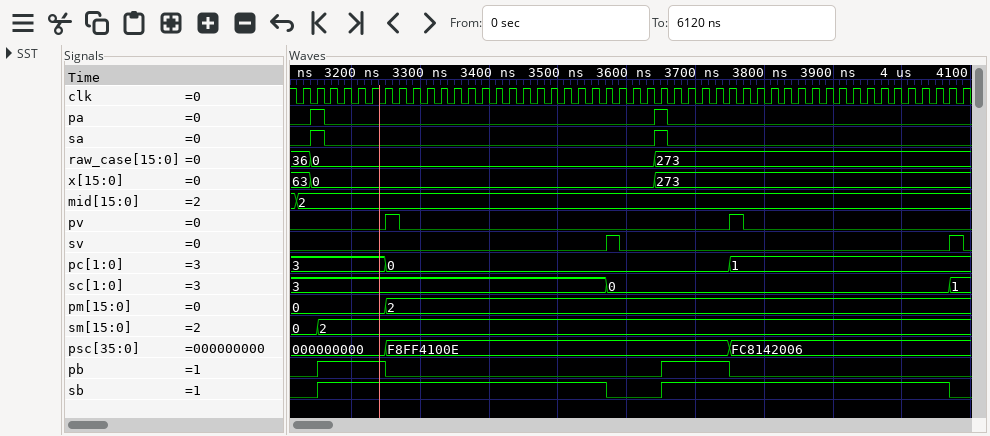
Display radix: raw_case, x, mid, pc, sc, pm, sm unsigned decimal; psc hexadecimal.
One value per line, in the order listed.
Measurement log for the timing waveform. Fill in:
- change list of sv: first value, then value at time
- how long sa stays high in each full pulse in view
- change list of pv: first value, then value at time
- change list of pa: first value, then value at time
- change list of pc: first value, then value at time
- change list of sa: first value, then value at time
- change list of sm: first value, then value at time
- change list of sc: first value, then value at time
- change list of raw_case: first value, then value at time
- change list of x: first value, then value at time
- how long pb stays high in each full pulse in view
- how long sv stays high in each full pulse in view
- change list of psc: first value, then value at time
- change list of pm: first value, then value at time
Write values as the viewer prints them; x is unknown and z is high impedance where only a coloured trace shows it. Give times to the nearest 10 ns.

0, 1 at 3570 ns, 0 at 3590 ns, 1 at 4070 ns, 0 at 4090 ns
20 ns, 20 ns
0, 1 at 3250 ns, 0 at 3270 ns, 1 at 3750 ns, 0 at 3770 ns
0, 1 at 3140 ns, 0 at 3160 ns, 1 at 3640 ns, 0 at 3660 ns
3, 0 at 3250 ns, 1 at 3750 ns
0, 1 at 3140 ns, 0 at 3160 ns, 1 at 3640 ns, 0 at 3660 ns
0, 2 at 3150 ns
3, 0 at 3570 ns, 1 at 4070 ns
36, 0 at 3140 ns, 273 at 3640 ns
63, 0 at 3140 ns, 273 at 3640 ns
100 ns, 100 ns
20 ns, 20 ns
000000000, F8FF4100E at 3250 ns, FC8142006 at 3750 ns
0, 2 at 3250 ns
